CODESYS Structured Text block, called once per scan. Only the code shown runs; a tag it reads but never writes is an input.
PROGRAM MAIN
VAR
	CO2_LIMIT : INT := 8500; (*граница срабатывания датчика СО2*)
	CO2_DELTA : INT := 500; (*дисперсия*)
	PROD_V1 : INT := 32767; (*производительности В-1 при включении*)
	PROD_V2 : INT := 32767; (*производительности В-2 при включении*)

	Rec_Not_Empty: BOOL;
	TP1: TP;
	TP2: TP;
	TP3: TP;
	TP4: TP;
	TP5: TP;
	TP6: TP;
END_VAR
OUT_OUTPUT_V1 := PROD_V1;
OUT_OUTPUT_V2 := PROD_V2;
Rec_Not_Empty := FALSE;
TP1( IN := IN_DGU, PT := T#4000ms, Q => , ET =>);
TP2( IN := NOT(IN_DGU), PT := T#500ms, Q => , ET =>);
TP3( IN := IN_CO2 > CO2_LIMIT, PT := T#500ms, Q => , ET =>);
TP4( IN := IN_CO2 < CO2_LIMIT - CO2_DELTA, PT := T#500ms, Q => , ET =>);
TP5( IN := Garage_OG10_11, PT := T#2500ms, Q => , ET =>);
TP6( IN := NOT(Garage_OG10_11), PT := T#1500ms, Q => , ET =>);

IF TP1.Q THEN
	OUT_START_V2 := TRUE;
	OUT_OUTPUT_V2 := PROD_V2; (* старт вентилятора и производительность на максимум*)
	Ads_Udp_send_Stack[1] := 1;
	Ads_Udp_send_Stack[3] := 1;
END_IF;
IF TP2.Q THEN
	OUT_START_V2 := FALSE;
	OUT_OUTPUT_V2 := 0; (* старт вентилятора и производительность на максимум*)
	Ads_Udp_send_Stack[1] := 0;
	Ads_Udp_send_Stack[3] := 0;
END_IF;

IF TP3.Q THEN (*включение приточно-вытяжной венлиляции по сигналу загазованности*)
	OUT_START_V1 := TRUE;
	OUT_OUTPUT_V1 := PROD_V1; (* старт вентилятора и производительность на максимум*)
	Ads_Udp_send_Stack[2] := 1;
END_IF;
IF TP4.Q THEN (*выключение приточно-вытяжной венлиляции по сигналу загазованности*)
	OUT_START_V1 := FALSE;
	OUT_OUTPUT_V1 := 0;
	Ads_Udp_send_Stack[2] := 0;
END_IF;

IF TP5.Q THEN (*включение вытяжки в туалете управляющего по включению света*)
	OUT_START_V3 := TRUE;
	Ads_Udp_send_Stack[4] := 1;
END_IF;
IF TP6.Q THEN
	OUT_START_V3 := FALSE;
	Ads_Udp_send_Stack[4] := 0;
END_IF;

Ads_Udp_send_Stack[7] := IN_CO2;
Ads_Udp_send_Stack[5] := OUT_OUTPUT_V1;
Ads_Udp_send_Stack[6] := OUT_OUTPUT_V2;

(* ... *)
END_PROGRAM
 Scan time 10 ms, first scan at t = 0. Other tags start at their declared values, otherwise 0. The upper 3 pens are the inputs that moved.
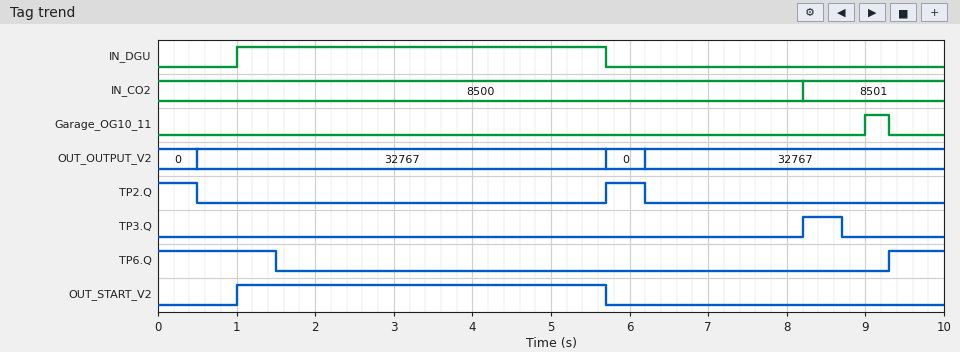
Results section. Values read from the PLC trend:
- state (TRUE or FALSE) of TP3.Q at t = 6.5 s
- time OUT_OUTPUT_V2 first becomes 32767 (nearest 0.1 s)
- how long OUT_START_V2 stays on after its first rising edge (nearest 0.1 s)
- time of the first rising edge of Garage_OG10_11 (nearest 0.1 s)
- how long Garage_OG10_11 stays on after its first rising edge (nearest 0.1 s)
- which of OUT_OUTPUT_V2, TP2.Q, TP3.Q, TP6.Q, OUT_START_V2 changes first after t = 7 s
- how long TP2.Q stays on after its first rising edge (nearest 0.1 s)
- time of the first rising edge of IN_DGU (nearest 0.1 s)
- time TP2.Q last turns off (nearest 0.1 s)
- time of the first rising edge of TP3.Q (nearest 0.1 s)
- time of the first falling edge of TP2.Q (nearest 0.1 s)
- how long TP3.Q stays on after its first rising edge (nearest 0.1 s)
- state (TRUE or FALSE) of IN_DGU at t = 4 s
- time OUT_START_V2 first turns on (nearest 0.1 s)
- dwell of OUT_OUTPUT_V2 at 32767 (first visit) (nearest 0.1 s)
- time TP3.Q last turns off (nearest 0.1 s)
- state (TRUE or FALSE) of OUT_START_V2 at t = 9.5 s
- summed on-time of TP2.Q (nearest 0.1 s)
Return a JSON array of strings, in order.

["FALSE", "0.5 s", "4.7 s", "9.0 s", "0.3 s", "TP3.Q", "0.5 s", "1.0 s", "6.2 s", "8.2 s", "0.5 s", "0.5 s", "TRUE", "1.0 s", "5.2 s", "8.7 s", "FALSE", "1.0 s"]
